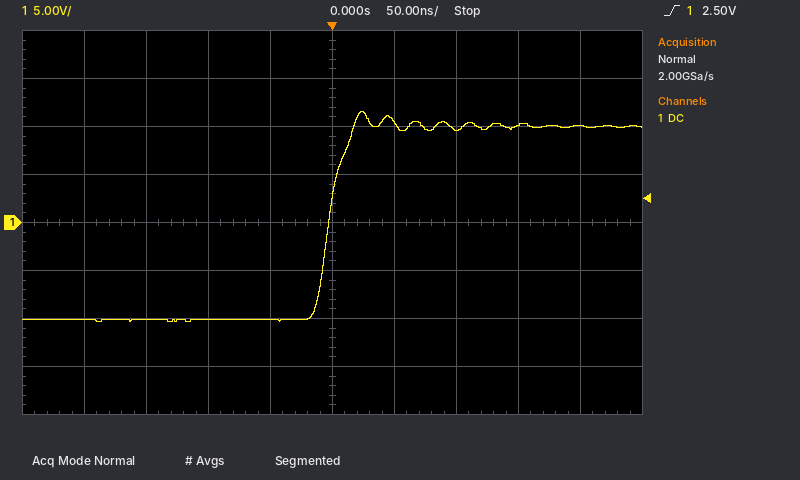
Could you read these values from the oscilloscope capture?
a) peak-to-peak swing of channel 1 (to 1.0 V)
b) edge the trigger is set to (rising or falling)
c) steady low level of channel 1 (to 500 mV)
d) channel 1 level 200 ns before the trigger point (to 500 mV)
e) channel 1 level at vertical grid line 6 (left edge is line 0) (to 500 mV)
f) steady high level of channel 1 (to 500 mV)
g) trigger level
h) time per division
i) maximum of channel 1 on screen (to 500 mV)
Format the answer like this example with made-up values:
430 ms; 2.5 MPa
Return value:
22.0 V; rising; -10.0 V; -10.0 V; 10.5 V; 10.0 V; 2.50 V; 50 ns; 11.5 V
